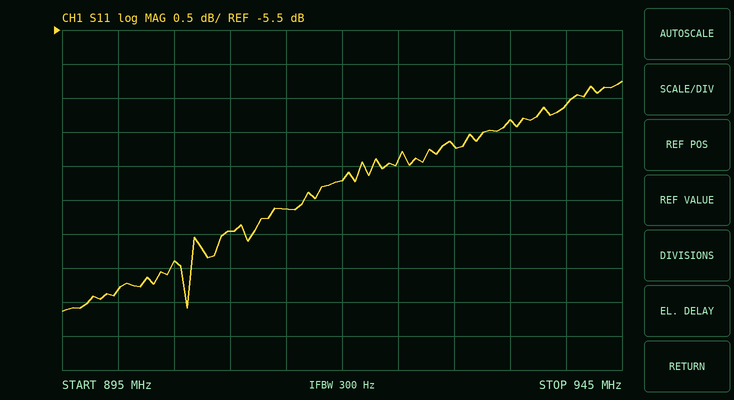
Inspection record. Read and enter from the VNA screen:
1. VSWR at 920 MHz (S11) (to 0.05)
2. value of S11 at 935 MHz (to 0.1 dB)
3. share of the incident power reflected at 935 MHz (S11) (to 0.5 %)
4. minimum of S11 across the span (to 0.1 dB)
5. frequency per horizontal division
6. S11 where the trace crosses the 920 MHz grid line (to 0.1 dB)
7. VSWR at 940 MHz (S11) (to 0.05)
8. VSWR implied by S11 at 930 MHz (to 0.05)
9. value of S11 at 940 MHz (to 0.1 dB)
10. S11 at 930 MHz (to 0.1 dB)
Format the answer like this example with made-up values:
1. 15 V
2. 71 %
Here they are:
1. 2.40
2. -6.8 dB
3. 21.0 %
4. -9.6 dB
5. 5 MHz
6. -7.7 dB
7. 2.75
8. 2.55
9. -6.6 dB
10. -7.2 dB
